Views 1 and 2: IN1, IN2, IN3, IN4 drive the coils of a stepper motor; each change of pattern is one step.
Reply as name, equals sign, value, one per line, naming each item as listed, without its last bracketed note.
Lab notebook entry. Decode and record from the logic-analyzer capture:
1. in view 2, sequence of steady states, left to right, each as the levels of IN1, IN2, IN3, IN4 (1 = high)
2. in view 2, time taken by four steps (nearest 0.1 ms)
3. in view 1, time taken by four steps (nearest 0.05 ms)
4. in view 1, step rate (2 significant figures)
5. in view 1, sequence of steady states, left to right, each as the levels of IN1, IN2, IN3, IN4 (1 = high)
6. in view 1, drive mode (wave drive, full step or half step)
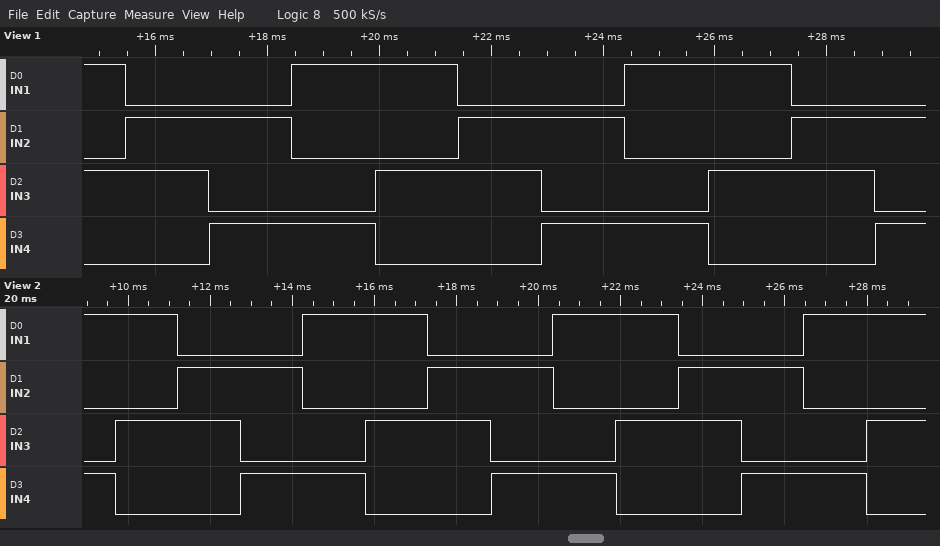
in view 2, sequence of steady states, left to right, each as the levels of IN1, IN2, IN3, IN4 = 1001 1010 0110 0101 1001 1010 0110 0101 1001 1010 0110 0101 1001 1010
in view 2, time taken by four steps = 6.1 ms
in view 1, time taken by four steps = 5.95 ms
in view 1, step rate = 670 steps/s
in view 1, sequence of steady states, left to right, each as the levels of IN1, IN2, IN3, IN4 = 1010 0110 0101 1001 1010 0110 0101 1001 1010 0110 0101
in view 1, drive mode = full step
